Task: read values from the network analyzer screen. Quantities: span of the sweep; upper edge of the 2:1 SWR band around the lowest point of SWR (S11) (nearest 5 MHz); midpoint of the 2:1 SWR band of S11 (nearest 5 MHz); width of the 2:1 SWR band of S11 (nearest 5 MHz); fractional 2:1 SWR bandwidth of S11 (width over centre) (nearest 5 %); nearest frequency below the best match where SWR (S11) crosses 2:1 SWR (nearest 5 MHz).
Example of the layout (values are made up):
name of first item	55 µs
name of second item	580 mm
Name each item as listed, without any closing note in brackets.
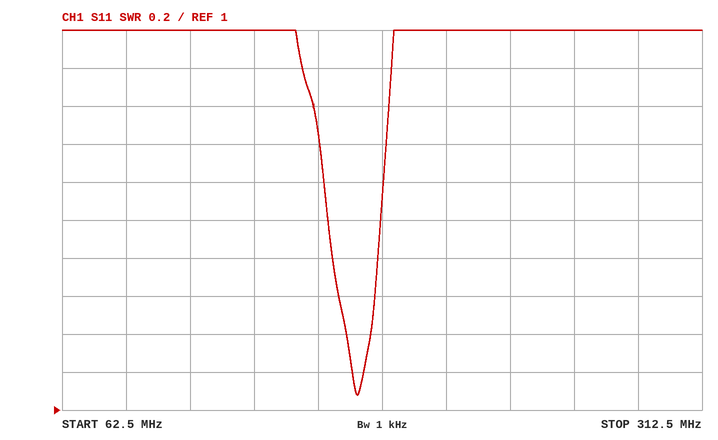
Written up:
span of the sweep	250 MHz
upper edge of the 2:1 SWR band around the lowest point of SWR (S11)	185 MHz
midpoint of the 2:1 SWR band of S11	175 MHz
width of the 2:1 SWR band of S11	20 MHz
fractional 2:1 SWR bandwidth of S11 (width over centre)	10 %
nearest frequency below the best match where SWR (S11) crosses 2:1 SWR	165 MHz
